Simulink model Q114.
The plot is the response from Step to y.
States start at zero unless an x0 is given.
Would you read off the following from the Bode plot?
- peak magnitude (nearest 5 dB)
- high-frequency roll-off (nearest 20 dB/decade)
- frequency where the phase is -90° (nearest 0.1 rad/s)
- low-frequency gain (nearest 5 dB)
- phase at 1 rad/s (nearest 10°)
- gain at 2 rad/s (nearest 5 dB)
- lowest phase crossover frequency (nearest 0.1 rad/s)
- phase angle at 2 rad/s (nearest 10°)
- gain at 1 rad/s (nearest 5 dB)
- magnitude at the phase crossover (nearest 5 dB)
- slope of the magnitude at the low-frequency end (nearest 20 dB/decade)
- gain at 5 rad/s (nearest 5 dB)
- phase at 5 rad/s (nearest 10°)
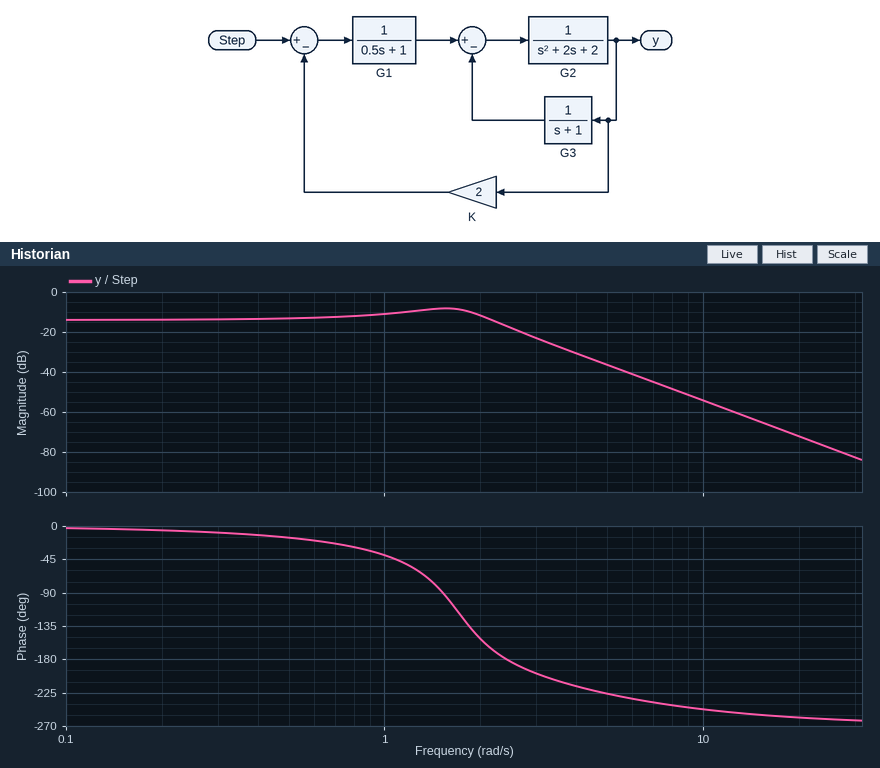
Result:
-10 dB
-60 dB/decade
1.5 rad/s
-15 dB
-40°
-10 dB
2.4 rad/s
-150°
-10 dB
-15 dB
0 dB/decade
-35 dB
-230°
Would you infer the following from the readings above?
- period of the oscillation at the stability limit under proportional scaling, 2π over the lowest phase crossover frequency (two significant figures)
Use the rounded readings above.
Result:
2.6 s
